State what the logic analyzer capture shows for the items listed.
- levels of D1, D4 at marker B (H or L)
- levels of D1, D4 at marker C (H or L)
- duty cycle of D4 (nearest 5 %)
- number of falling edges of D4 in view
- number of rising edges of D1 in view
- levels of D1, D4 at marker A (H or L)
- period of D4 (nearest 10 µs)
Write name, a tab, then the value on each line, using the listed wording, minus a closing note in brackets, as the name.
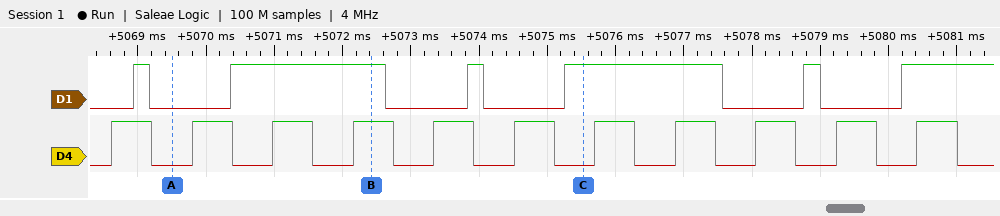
levels of D1, D4 at marker B	D1=H, D4=H
levels of D1, D4 at marker C	D1=H, D4=L
duty cycle of D4	50 %
number of falling edges of D4 in view	11
number of rising edges of D1 in view	6
levels of D1, D4 at marker A	D1=L, D4=L
period of D4	1180 µs
